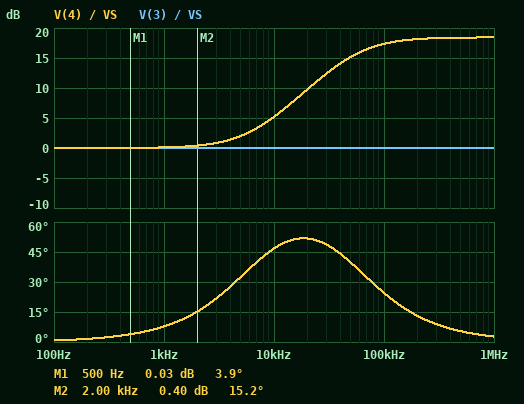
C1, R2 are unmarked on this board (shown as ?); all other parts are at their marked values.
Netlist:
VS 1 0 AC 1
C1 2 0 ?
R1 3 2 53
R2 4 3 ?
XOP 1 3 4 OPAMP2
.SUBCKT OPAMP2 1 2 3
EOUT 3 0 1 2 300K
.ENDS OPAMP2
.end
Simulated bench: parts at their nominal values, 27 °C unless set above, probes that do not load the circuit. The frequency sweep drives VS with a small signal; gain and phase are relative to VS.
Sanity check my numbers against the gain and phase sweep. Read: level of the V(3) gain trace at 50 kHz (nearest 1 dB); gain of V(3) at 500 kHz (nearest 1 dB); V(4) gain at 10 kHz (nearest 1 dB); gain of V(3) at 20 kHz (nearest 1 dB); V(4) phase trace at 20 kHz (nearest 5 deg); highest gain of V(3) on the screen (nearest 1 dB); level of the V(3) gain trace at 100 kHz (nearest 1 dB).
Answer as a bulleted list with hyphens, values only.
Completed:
- 0 dB
- 0 dB
- 5 dB
- 0 dB
- 50 deg
- 0 dB
- 0 dB
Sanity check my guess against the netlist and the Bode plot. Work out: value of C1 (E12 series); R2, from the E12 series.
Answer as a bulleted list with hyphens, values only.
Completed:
- 56 nF
- 390 Ω
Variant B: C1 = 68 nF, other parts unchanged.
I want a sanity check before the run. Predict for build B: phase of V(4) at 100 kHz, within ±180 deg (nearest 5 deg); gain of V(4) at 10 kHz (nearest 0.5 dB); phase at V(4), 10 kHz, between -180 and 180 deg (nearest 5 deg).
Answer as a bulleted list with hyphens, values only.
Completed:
- 20 deg
- 6.5 dB
- 50 deg
